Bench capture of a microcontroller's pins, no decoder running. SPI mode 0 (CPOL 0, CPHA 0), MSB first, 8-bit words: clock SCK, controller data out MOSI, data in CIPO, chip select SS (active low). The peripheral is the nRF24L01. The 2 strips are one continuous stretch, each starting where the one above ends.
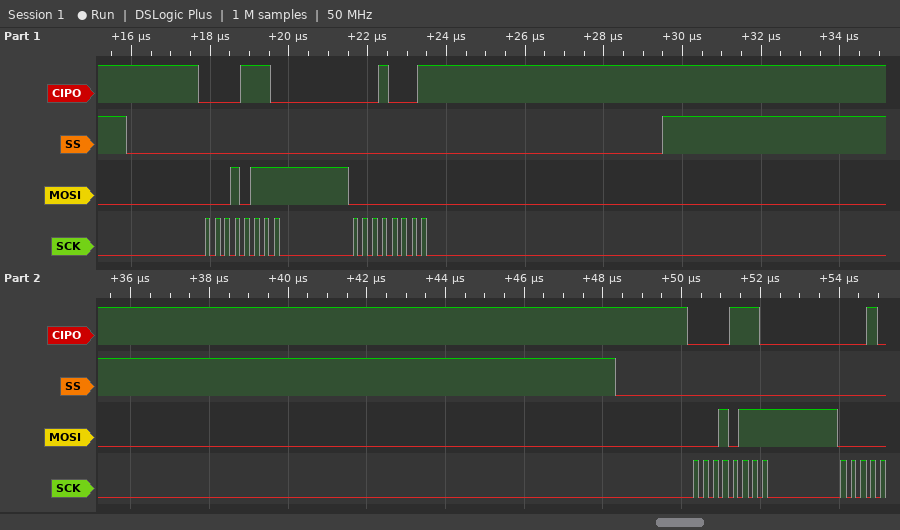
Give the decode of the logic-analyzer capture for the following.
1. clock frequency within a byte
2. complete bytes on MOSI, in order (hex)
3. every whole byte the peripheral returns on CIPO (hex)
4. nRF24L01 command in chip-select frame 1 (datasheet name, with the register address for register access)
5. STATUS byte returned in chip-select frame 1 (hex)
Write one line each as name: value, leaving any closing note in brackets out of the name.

clock frequency within a byte: 4 MHz
complete bytes on MOSI, in order: 17 00 17
every whole byte the peripheral returns on CIPO: 0E 11 0E
nRF24L01 command in chip-select frame 1: R_REGISTER 0x17
STATUS byte returned in chip-select frame 1: 0x0E
